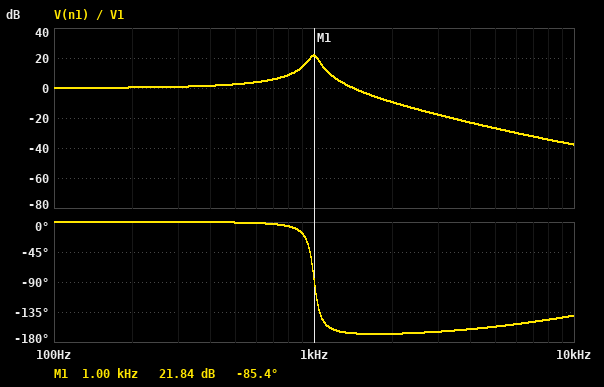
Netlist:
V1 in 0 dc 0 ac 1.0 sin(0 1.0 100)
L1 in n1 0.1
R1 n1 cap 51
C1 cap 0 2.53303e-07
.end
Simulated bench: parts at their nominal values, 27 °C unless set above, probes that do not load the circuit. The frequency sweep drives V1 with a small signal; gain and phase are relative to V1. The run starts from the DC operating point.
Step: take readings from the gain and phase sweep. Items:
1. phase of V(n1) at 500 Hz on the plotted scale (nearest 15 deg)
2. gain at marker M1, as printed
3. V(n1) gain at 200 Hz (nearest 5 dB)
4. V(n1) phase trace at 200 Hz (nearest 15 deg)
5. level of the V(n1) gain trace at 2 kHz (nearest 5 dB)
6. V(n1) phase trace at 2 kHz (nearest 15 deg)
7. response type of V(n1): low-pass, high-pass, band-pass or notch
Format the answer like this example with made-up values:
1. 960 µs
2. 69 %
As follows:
1. 0 deg
2. 21.84 dB
3. 0 dB
4. 0 deg
5. -10 dB
6. -165 deg
7. low-pass
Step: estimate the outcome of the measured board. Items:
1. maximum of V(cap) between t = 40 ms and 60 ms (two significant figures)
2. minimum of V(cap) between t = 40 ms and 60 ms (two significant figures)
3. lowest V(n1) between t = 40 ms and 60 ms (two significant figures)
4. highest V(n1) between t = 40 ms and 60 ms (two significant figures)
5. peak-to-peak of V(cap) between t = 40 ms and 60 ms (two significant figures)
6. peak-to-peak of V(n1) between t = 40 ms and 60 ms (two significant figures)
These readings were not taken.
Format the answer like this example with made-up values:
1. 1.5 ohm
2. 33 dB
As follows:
1. 1.0 V
2. -1.0 V
3. -1.0 V
4. 1.0 V
5. 2.0 V
6. 2.0 V
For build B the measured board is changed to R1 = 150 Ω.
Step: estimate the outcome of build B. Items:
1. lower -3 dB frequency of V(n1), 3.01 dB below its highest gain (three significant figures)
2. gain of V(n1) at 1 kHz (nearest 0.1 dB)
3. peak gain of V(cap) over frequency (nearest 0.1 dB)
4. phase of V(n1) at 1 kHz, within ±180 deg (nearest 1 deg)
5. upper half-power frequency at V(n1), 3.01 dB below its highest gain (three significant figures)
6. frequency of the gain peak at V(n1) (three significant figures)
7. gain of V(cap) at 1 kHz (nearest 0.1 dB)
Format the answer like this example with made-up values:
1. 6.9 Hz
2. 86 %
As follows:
1. 859 Hz
2. 12.7 dB
3. 12.5 dB
4. -77 deg
5. 1.10 kHz
6. 986 Hz
7. 12.4 dB
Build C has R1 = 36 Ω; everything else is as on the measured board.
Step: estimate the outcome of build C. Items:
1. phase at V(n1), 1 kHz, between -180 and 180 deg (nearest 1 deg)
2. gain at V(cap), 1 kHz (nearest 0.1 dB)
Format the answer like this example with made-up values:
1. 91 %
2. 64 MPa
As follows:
1. -87 deg
2. 24.8 dB
